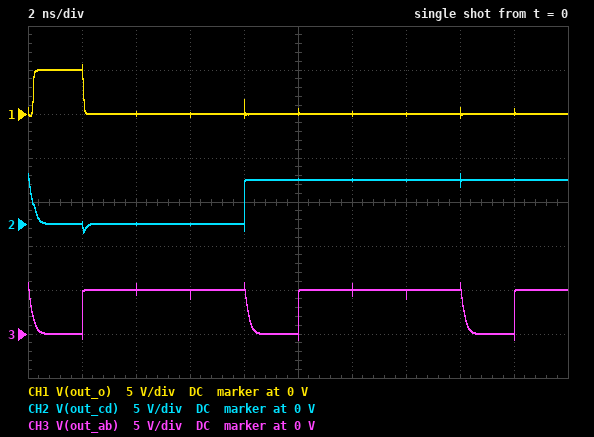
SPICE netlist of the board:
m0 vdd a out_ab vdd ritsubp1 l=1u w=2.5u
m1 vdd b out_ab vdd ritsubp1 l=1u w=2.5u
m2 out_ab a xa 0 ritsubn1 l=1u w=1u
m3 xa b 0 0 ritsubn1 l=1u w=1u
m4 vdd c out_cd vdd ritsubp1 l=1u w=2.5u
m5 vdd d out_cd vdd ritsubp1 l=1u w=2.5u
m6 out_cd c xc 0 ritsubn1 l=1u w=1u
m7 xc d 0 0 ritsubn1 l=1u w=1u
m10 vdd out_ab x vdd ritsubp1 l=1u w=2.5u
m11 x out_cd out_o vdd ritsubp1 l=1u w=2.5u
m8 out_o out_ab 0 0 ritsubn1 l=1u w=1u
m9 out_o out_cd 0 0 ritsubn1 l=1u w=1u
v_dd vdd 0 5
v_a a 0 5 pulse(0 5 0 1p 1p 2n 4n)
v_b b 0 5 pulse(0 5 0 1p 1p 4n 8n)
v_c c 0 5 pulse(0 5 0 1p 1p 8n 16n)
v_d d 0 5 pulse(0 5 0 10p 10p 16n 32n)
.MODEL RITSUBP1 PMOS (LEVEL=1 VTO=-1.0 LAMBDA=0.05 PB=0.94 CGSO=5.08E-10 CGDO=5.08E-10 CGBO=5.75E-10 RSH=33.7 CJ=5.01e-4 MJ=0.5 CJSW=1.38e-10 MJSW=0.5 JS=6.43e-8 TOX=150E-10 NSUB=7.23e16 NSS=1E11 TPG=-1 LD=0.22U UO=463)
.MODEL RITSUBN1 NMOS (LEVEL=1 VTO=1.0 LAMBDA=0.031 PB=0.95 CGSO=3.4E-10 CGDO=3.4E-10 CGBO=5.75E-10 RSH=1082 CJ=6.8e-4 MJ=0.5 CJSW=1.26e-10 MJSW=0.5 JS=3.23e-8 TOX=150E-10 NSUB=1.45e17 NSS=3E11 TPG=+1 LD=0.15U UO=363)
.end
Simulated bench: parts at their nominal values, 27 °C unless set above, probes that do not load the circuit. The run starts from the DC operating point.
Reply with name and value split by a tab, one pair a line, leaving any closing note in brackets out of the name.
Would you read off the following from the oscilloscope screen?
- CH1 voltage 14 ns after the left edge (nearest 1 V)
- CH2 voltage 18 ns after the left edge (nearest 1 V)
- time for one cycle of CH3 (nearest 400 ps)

CH1 voltage 14 ns after the left edge	0 V
CH2 voltage 18 ns after the left edge	5 V
time for one cycle of CH3	8.0 ns
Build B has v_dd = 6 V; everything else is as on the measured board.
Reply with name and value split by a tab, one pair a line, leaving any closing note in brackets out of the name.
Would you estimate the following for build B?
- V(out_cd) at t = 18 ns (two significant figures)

V(out_cd) at t = 18 ns	6.0 V
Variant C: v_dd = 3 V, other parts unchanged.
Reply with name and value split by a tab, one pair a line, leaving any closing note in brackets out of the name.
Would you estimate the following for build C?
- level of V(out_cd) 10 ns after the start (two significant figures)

level of V(out_cd) 10 ns after the start	3.0 V
